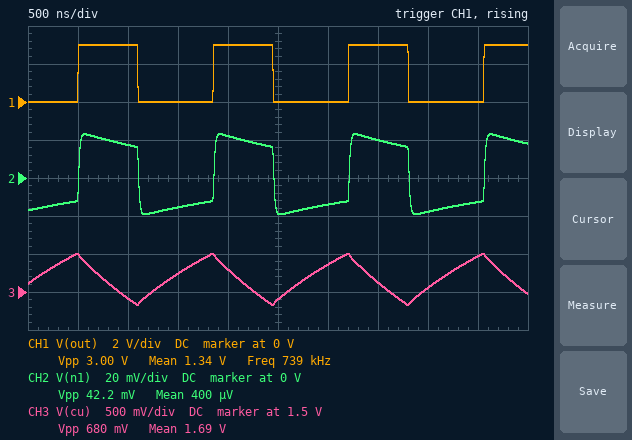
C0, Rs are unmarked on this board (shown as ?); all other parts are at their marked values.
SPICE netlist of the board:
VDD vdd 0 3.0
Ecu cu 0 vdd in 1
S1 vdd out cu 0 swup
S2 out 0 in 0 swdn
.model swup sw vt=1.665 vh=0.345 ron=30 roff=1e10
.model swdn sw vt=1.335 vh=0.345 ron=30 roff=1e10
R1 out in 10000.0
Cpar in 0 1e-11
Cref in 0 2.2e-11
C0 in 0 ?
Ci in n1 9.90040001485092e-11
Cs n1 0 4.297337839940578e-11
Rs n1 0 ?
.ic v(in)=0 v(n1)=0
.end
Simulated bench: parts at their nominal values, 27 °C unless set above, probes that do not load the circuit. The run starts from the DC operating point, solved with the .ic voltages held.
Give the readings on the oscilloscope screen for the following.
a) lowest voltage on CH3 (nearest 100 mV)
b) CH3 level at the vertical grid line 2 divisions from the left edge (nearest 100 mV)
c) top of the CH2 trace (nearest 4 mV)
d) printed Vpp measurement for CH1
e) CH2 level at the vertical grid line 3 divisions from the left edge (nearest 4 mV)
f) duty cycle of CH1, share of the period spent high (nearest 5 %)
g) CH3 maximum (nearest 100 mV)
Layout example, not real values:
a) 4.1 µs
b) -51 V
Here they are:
a) 1.3 V
b) 1.4 V
c) 24 mV
d) 3.00 V
e) -16 mV
f) 45 %
g) 2.0 V
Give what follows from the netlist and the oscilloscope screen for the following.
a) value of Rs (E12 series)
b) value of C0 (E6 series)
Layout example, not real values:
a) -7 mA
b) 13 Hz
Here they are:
a) 180 Ω
b) 15 pF
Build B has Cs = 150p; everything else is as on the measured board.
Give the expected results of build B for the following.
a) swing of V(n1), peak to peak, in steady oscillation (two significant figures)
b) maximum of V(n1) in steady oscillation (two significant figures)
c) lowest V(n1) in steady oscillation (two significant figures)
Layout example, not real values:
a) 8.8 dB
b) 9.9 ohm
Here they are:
a) 40 mV
b) 22 mV
c) -18 mV
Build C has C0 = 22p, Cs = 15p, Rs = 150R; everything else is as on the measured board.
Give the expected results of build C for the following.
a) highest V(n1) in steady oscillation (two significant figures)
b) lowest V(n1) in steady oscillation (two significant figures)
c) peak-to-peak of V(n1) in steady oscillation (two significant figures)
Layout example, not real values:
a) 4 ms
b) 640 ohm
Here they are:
a) 19 mV
b) -16 mV
c) 34 mV
